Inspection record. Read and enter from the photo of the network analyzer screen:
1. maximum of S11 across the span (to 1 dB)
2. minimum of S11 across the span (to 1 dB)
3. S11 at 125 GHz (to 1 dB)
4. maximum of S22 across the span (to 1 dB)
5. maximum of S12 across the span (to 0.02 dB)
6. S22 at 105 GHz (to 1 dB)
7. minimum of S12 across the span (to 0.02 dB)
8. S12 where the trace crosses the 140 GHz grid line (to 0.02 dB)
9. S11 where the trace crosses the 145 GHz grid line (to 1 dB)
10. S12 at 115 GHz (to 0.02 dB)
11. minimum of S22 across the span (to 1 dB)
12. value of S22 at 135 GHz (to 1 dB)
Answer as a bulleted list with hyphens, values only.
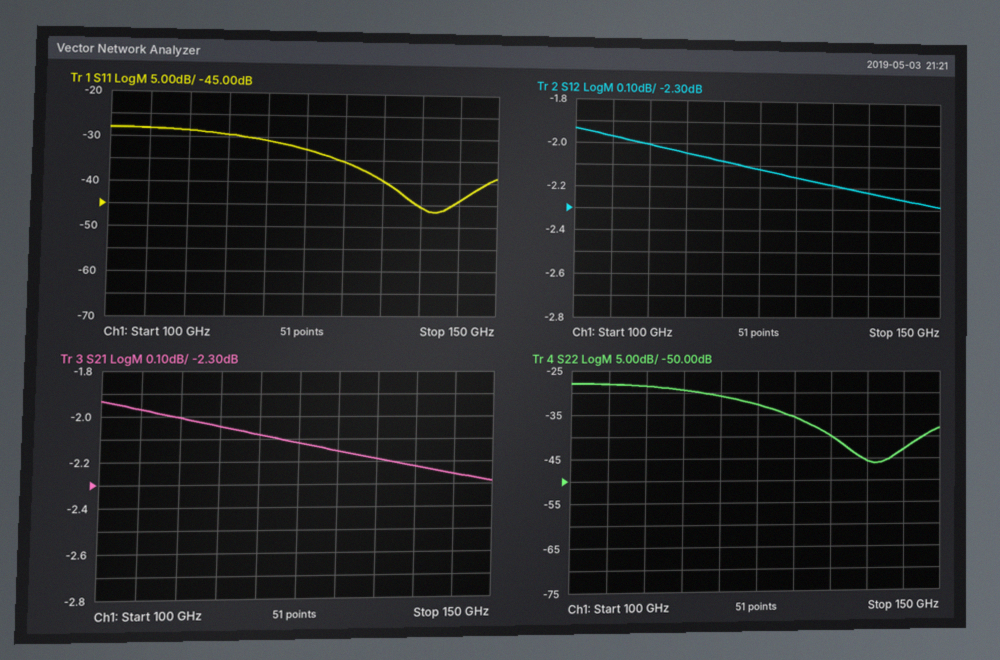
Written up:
- -28 dB
- -47 dB
- -33 dB
- -28 dB
- -1.94 dB
- -28 dB
- -2.28 dB
- -2.22 dB
- -44 dB
- -2.04 dB
- -46 dB
- -40 dB
